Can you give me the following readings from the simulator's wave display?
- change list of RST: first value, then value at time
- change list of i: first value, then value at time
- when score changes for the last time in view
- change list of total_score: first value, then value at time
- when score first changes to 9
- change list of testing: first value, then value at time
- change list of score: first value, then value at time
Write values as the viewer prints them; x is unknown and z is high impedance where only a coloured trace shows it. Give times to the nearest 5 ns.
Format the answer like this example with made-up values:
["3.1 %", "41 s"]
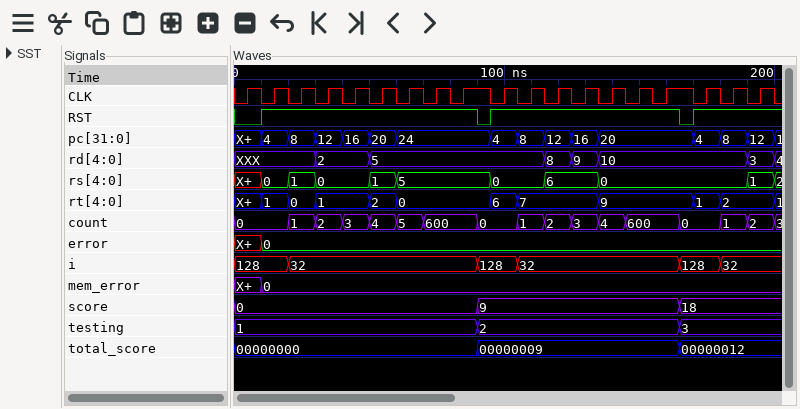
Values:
["0, 1 at 10 ns, 0 at 90 ns, 1 at 95 ns, 0 at 165 ns, 1 at 170 ns", "128, 32 at 20 ns, 128 at 90 ns, 32 at 105 ns, 128 at 165 ns, 32 at 180 ns", "165 ns", "00000000, 00000009 at 90 ns, 00000012 at 165 ns", "90 ns", "1, 2 at 90 ns, 3 at 165 ns", "0, 9 at 90 ns, 18 at 165 ns"]
